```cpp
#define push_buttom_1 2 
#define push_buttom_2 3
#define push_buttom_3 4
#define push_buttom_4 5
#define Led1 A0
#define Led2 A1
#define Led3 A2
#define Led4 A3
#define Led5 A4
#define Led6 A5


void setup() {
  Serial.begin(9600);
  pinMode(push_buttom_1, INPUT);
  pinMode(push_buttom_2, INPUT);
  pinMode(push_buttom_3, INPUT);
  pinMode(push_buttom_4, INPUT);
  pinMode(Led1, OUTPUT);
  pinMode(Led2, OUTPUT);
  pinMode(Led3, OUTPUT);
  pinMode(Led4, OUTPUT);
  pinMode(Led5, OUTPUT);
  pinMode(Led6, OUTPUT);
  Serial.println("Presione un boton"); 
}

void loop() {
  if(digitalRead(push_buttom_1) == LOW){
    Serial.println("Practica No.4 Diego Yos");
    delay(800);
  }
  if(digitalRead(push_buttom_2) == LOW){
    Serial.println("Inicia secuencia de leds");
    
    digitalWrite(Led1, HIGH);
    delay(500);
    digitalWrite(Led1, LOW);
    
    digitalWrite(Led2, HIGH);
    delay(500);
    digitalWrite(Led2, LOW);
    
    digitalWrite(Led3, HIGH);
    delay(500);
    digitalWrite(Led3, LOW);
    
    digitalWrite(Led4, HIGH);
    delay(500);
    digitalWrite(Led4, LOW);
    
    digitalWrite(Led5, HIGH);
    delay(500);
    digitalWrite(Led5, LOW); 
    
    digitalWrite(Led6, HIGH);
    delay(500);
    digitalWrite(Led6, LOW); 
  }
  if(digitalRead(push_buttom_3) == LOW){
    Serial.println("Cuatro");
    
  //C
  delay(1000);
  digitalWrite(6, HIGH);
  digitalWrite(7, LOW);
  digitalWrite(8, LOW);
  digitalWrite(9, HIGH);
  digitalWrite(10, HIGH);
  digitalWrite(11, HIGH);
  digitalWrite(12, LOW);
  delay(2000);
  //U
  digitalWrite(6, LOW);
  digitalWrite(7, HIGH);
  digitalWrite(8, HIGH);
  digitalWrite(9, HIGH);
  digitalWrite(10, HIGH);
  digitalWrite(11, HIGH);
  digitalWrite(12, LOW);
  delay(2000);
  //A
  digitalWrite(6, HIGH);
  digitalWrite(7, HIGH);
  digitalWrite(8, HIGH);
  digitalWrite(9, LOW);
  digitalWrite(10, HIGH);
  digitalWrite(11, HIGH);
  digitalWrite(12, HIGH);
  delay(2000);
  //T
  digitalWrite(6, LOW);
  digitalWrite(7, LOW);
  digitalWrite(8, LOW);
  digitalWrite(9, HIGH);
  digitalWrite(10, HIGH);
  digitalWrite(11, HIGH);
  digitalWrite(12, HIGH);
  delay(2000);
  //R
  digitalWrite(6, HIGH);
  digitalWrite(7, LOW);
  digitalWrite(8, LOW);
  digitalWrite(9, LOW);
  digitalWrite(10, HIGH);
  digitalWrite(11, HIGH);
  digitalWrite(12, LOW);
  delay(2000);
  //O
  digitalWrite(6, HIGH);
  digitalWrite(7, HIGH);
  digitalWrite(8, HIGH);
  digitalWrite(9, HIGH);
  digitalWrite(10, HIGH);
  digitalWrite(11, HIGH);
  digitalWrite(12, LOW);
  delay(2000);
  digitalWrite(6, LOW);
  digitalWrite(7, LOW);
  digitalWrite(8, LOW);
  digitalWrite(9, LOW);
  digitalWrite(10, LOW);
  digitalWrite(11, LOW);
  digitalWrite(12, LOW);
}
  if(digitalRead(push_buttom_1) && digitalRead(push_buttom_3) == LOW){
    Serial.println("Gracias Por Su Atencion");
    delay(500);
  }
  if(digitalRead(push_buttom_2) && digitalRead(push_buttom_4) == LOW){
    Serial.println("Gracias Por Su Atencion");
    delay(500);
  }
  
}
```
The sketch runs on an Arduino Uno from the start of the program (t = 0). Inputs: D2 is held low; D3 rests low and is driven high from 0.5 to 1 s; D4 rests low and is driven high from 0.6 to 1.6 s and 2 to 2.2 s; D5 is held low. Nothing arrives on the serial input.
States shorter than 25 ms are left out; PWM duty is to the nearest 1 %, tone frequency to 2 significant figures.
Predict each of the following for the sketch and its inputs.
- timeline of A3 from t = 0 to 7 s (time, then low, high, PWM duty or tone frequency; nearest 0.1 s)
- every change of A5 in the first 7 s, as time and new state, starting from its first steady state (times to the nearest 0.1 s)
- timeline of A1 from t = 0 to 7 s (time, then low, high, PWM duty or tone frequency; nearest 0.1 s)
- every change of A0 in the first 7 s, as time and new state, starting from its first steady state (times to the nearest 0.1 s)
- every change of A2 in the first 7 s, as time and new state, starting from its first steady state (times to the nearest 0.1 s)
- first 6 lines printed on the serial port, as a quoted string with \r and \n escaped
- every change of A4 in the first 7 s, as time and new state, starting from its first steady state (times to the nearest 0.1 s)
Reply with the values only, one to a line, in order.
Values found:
0 s low; 3.6 s high; 4.1 s low
0 s low; 4.6 s high; 5.1 s low
0 s low; 2.6 s high; 3.1 s low
0 s low; 2.1 s high; 2.6 s low
0 s low; 3.1 s high; 3.6 s low
"Presione un boton\r\nPractica No.4 Diego Yos\r\nGracias Por Su Atencion\r\nPractica No.4 Diego Yos\r\nInicia secuencia de leds\r\nCuatro\r\n"
0 s low; 4.1 s high; 4.6 s low
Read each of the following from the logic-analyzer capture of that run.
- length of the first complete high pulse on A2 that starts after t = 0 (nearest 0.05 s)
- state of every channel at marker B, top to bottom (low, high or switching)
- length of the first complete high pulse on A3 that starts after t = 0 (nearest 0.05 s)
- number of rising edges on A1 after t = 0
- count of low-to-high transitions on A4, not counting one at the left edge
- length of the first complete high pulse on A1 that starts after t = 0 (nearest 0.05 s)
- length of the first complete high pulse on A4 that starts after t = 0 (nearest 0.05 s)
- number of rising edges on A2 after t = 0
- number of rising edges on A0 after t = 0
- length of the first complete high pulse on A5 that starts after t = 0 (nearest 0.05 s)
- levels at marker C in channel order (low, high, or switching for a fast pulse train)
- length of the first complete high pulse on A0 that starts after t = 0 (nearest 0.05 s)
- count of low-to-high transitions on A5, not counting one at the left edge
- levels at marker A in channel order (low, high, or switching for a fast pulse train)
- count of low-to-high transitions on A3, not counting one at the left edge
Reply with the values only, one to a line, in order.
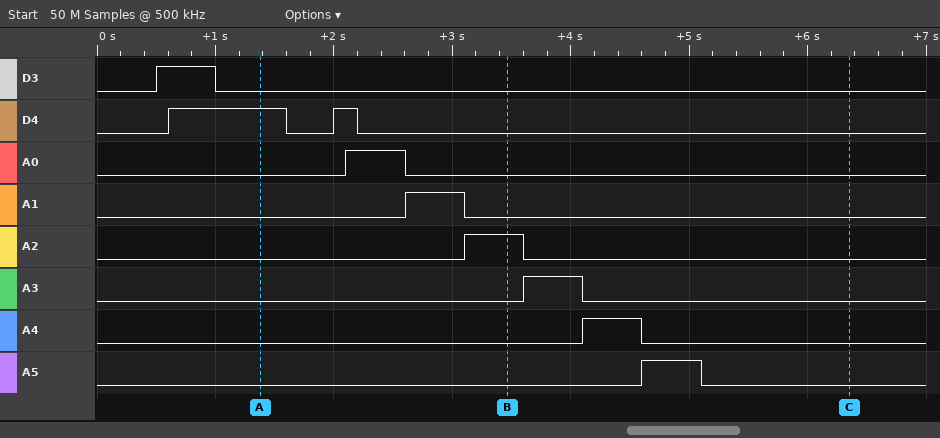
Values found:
0.50 s
D3 low, D4 low, A0 low, A1 low, A2 high, A3 low, A4 low, A5 low
0.50 s
1
1
0.50 s
0.50 s
1
1
0.50 s
D3 low, D4 low, A0 low, A1 low, A2 low, A3 low, A4 low, A5 low
0.50 s
1
D3 low, D4 high, A0 low, A1 low, A2 low, A3 low, A4 low, A5 low
1
